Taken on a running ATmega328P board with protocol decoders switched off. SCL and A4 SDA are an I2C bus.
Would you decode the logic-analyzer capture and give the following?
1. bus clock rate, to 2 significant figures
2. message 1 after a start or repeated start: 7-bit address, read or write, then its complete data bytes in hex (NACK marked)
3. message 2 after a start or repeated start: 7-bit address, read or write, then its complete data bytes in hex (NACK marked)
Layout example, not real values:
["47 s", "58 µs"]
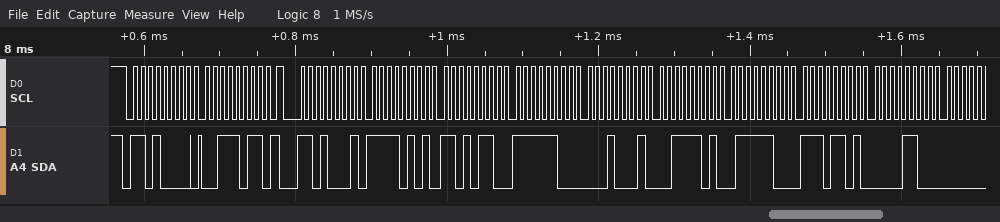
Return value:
["100 kHz", "0x68 write: 3B", "0x68 read: F5 D6 FC 11 3D 7C ED 0C"]
